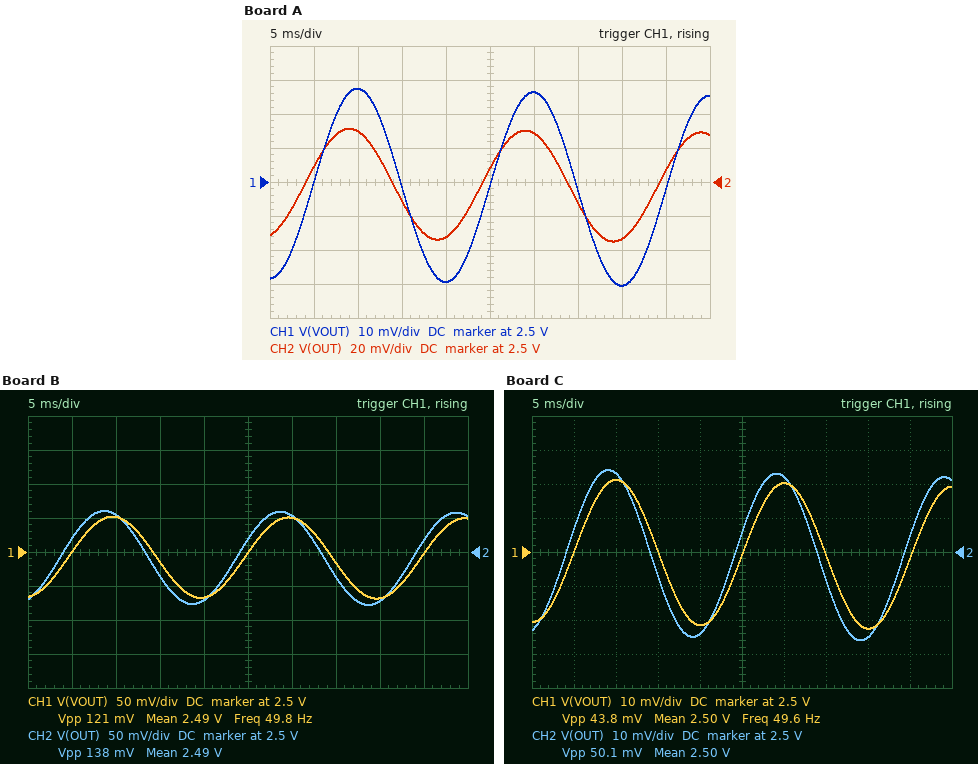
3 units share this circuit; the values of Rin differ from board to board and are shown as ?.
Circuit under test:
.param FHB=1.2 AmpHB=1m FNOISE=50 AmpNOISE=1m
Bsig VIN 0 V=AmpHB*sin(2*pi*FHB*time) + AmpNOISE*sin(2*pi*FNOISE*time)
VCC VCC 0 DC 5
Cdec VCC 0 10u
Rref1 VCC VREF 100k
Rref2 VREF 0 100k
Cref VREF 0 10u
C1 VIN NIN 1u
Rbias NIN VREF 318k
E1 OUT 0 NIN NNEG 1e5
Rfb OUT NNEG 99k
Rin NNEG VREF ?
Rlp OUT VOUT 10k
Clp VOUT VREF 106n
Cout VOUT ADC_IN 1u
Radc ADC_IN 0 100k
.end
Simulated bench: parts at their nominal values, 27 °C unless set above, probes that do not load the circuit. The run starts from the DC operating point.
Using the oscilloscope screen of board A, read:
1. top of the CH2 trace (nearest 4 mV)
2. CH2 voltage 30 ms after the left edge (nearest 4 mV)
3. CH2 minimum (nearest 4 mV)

2.532 V
2.528 V
2.464 V
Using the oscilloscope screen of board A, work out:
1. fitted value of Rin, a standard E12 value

2.2 kΩ
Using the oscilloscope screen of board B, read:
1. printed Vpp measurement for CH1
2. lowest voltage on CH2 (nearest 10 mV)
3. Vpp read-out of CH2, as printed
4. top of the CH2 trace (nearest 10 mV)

121 mV
2.42 V
138 mV
2.56 V
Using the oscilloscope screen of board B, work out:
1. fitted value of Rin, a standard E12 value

470 Ω
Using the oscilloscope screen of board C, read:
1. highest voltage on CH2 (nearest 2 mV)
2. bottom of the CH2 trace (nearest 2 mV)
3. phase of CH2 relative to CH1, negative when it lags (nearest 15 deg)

2.524 V
2.474 V
15 deg
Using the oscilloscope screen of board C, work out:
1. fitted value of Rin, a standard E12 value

3.3 kΩ
